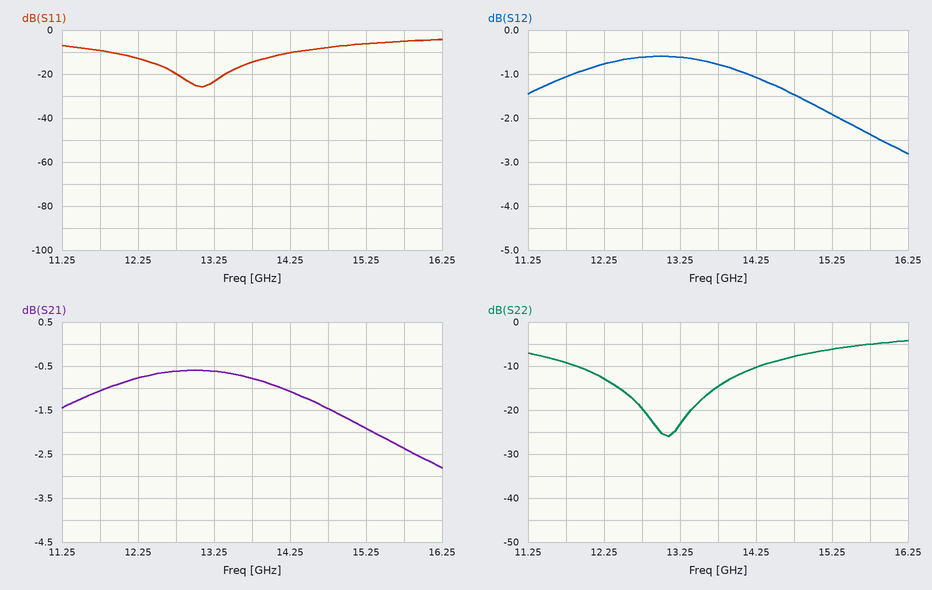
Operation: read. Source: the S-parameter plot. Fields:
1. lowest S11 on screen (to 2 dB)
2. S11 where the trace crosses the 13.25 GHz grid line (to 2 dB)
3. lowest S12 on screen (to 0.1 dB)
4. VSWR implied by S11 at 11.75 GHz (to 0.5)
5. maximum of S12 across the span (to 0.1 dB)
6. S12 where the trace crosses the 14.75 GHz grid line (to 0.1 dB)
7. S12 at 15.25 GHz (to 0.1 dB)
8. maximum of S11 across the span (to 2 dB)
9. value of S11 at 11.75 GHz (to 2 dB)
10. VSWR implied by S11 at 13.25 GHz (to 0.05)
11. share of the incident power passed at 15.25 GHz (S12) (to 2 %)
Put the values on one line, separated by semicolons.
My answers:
-26 dB; -24 dB; -2.8 dB; 2.0; -0.6 dB; -1.5 dB; -1.9 dB; -4 dB; -10 dB; 1.15; 64 %
